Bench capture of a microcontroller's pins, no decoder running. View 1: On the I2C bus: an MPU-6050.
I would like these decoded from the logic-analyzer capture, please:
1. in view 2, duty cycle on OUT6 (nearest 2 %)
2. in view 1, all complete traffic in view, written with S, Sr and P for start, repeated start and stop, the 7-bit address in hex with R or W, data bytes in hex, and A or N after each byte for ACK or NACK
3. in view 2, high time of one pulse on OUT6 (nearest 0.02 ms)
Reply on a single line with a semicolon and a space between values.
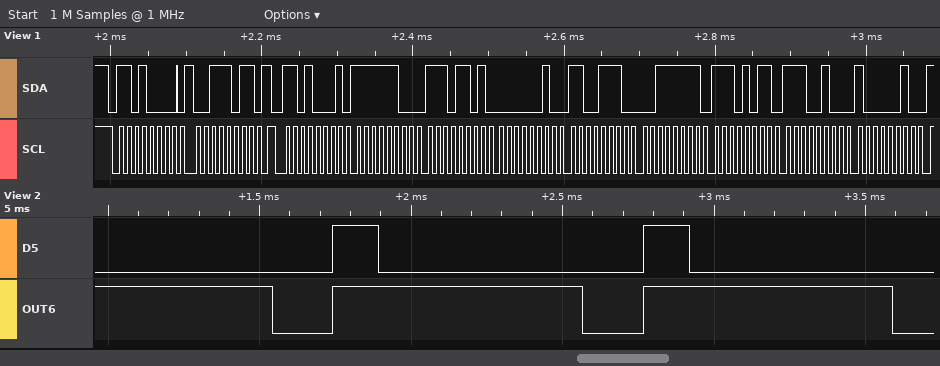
80 %; S 68W A 3B A Sr 68R A FC A ED A 02 A CE A 3F A EB A E4 A 82 A; 0.82 ms
